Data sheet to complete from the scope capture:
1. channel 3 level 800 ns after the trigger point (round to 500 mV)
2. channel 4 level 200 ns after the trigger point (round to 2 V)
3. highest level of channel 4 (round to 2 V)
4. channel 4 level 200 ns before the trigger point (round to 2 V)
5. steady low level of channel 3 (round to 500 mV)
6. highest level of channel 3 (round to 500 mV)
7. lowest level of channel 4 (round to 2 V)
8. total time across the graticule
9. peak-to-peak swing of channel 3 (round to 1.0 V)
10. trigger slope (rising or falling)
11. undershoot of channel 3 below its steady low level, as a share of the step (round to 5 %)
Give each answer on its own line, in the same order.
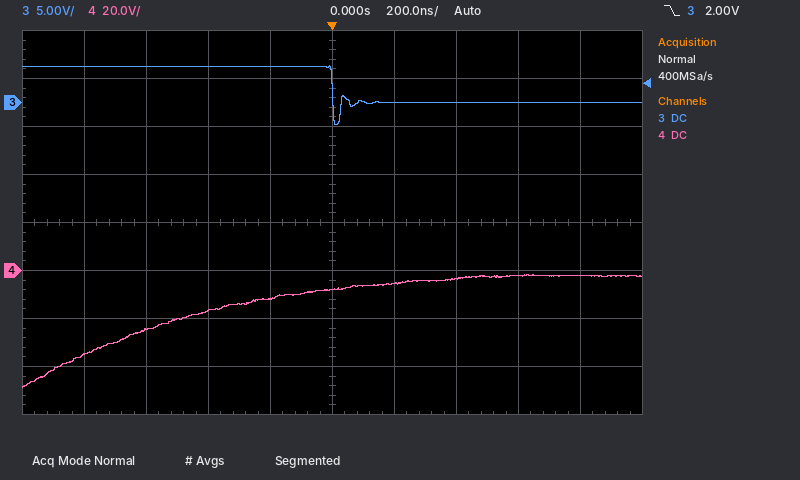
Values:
0.0 V
-6 V
-2 V
-12 V
0.0 V
4.0 V
-48 V
2 µs
6.0 V
falling
60 %
